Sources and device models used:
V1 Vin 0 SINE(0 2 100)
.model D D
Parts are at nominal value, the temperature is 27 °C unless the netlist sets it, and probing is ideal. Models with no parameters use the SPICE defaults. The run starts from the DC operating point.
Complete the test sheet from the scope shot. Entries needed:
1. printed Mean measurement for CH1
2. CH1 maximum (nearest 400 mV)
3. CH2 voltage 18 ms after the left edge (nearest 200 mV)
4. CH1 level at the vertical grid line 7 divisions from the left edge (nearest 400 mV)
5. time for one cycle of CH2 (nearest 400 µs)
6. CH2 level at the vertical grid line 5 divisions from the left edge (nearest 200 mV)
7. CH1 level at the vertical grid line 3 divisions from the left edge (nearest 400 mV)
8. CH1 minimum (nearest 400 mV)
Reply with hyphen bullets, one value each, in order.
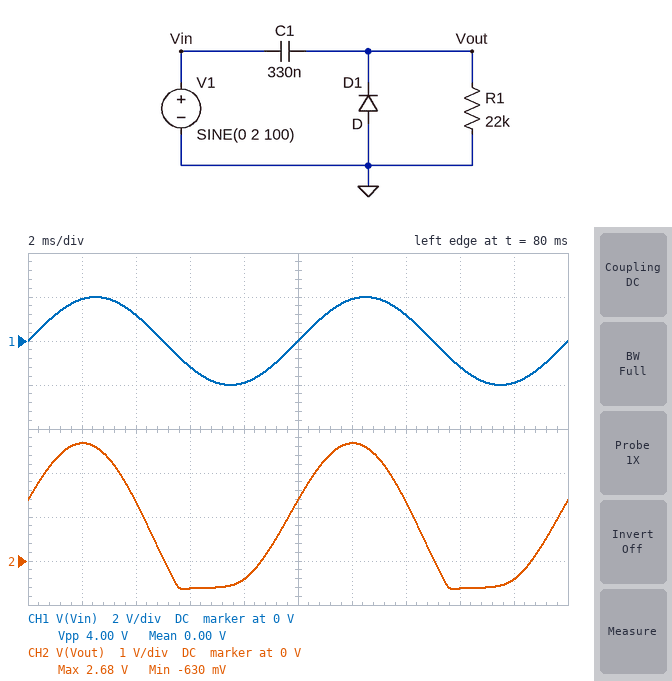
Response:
- 0.00 V
- 2.0 V
- -400 mV
- 1.2 V
- 10.0 ms
- 1.4 V
- -1.2 V
- -2.0 V
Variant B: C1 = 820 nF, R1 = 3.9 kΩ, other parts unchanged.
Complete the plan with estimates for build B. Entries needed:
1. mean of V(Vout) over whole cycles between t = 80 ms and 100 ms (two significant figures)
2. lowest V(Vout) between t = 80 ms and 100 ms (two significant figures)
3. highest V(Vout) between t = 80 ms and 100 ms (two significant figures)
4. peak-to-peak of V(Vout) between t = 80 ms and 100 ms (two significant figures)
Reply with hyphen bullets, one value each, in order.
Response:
- 530 mV
- -650 mV
- 2.1 V
- 2.7 V
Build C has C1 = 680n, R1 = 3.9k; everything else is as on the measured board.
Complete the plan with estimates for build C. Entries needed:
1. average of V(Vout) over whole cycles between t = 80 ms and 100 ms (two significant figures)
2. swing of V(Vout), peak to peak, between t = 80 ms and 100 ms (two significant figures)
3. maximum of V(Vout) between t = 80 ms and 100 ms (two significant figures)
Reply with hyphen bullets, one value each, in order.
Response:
- 450 mV
- 2.6 V
- 1.9 V
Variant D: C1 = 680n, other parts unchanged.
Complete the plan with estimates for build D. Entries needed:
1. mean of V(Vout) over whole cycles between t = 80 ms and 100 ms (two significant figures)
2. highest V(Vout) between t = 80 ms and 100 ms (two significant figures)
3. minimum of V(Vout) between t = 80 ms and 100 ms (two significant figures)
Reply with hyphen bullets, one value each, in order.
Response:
- 1.1 V
- 3.0 V
- -640 mV
